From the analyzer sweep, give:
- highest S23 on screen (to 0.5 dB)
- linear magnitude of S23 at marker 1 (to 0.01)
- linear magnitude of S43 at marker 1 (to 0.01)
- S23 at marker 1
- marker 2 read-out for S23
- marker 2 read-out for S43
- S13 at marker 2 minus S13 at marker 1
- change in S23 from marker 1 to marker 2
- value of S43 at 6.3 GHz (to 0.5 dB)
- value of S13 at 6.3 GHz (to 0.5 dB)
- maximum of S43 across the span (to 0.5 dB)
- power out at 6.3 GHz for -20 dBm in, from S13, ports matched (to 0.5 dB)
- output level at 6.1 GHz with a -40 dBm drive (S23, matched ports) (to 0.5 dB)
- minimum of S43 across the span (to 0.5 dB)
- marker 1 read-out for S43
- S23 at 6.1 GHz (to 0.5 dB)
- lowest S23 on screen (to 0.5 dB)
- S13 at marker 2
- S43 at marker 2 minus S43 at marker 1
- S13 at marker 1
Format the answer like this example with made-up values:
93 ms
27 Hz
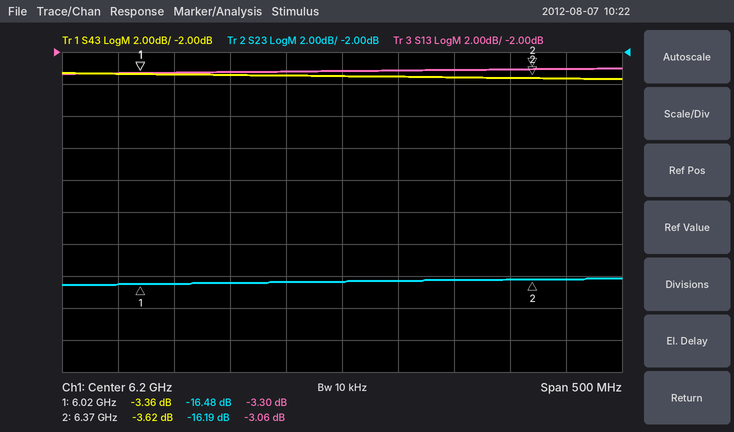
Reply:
-16.0 dB
0.15
0.68
-16.48 dB
-16.19 dB
-3.62 dB
0.24 dB
0.29 dB
-3.5 dB
-3.0 dB
-3.5 dB
-23.0 dBm
-56.5 dBm
-3.5 dB
-3.36 dB
-16.5 dB
-16.5 dB
-3.06 dB
-0.26 dB
-3.30 dB
